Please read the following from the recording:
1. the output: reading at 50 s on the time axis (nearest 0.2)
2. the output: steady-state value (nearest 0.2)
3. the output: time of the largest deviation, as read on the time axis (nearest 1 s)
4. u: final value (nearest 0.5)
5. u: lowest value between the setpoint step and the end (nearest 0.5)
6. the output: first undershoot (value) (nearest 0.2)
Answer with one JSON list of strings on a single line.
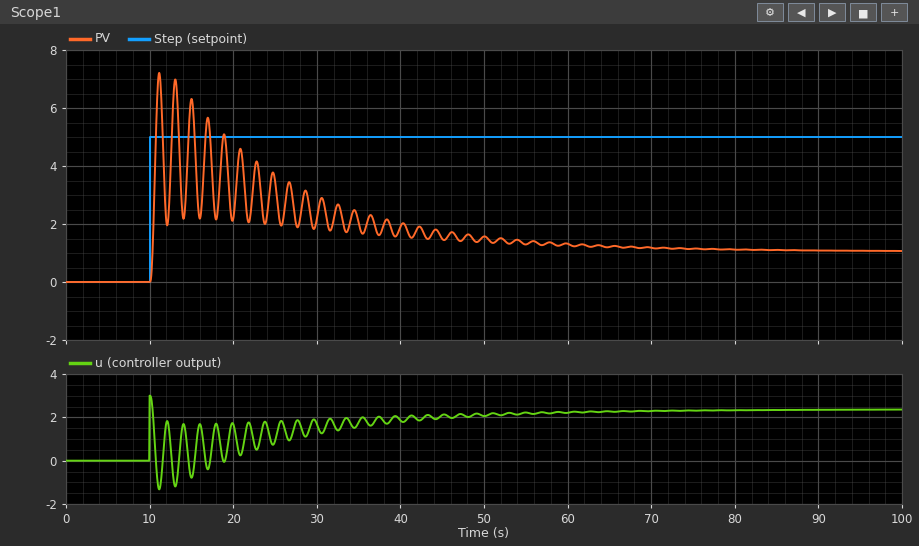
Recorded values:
["1.6", "1.0", "11 s", "2.5", "-1.5", "2.0"]
